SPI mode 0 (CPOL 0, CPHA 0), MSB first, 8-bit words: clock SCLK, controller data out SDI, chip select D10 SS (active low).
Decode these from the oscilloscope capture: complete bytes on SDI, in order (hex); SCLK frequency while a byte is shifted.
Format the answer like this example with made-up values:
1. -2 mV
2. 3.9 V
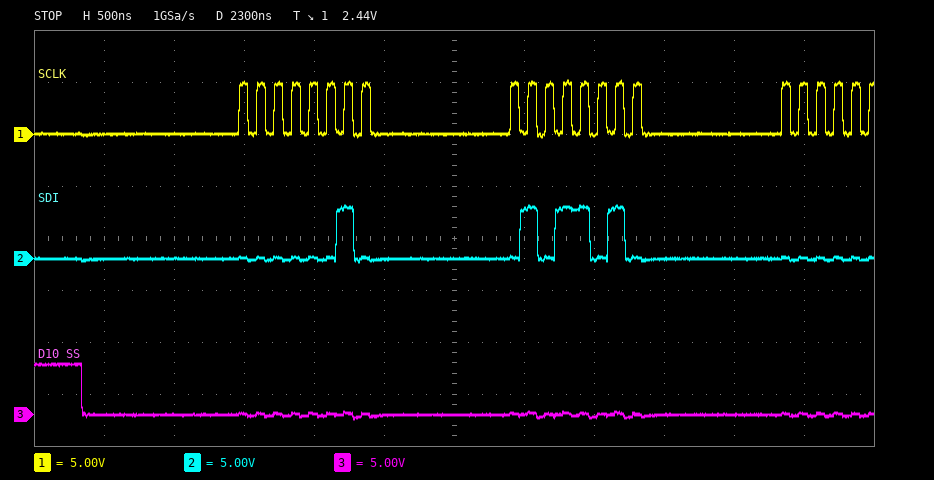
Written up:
1. 02 5A
2. 8 MHz
